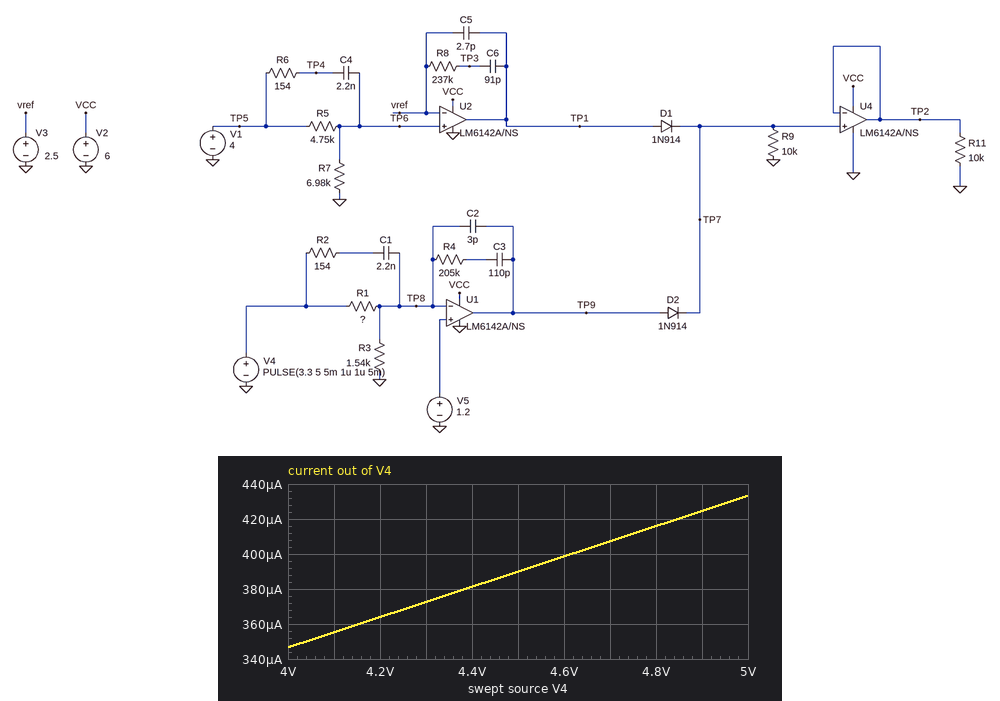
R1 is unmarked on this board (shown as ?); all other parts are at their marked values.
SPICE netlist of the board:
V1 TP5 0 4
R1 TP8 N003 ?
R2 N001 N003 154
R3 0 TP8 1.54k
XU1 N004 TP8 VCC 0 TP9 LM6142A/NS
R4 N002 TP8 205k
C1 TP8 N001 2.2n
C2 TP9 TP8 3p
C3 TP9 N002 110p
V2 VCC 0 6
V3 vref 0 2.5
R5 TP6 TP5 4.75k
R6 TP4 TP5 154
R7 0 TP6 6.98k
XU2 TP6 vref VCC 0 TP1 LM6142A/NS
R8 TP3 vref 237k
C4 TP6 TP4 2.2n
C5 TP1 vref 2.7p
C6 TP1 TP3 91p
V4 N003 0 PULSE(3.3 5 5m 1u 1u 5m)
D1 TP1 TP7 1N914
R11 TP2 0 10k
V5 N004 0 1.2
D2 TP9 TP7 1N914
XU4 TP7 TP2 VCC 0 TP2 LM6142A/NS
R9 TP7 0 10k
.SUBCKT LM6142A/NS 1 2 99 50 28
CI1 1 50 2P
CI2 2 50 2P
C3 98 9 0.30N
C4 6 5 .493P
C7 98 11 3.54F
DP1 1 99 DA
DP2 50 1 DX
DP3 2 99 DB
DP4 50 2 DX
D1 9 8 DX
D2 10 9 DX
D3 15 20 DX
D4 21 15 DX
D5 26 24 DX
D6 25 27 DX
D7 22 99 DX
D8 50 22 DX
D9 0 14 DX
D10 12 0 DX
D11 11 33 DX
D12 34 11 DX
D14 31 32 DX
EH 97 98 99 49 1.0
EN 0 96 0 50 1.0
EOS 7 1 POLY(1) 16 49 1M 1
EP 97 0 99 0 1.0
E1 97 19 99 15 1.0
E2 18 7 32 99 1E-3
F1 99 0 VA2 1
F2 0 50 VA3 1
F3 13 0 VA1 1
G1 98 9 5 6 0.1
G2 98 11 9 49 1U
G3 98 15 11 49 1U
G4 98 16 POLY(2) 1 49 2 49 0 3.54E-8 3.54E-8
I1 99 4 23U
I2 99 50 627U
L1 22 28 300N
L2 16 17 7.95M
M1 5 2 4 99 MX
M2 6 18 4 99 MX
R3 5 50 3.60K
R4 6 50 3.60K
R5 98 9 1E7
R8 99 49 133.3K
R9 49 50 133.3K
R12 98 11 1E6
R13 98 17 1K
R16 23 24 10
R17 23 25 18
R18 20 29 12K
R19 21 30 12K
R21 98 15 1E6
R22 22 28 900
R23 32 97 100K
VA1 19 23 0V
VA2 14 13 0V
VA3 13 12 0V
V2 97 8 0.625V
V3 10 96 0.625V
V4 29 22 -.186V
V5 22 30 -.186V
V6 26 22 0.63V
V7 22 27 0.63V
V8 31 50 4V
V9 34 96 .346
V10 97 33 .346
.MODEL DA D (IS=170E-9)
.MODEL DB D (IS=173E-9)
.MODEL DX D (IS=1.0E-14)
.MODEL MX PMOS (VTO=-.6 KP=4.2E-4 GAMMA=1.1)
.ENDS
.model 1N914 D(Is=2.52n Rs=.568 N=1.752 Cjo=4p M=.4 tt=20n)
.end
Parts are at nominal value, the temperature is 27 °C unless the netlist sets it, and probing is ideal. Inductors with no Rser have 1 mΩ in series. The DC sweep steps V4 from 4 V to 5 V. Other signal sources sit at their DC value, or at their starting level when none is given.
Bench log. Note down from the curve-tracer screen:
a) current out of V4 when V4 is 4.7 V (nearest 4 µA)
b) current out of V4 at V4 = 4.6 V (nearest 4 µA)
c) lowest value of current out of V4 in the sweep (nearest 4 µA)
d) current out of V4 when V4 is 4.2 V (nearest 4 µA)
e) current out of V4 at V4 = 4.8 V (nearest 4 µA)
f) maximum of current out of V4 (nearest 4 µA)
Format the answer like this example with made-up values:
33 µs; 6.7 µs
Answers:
408 µA; 400 µA; 348 µA; 364 µA; 416 µA; 432 µA
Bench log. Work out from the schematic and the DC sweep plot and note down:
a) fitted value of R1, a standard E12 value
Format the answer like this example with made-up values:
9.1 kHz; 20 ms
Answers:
10 kΩ
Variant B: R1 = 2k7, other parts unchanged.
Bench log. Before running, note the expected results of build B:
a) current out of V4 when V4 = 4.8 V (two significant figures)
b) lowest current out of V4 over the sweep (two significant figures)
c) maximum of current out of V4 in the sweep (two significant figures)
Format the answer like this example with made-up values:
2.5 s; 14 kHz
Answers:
1.1 mA; 940 µA; 1.2 mA
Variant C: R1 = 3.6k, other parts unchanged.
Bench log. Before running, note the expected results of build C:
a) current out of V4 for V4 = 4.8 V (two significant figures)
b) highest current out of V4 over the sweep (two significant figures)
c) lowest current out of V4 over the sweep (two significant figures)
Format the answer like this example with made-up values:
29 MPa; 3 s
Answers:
930 µA; 970 µA; 780 µA
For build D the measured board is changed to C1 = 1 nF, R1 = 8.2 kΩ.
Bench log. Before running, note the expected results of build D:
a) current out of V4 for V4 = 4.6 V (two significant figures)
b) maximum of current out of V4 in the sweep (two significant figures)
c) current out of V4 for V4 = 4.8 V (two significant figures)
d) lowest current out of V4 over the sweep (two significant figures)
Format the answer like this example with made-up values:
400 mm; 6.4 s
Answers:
470 µA; 510 µA; 490 µA; 410 µA
